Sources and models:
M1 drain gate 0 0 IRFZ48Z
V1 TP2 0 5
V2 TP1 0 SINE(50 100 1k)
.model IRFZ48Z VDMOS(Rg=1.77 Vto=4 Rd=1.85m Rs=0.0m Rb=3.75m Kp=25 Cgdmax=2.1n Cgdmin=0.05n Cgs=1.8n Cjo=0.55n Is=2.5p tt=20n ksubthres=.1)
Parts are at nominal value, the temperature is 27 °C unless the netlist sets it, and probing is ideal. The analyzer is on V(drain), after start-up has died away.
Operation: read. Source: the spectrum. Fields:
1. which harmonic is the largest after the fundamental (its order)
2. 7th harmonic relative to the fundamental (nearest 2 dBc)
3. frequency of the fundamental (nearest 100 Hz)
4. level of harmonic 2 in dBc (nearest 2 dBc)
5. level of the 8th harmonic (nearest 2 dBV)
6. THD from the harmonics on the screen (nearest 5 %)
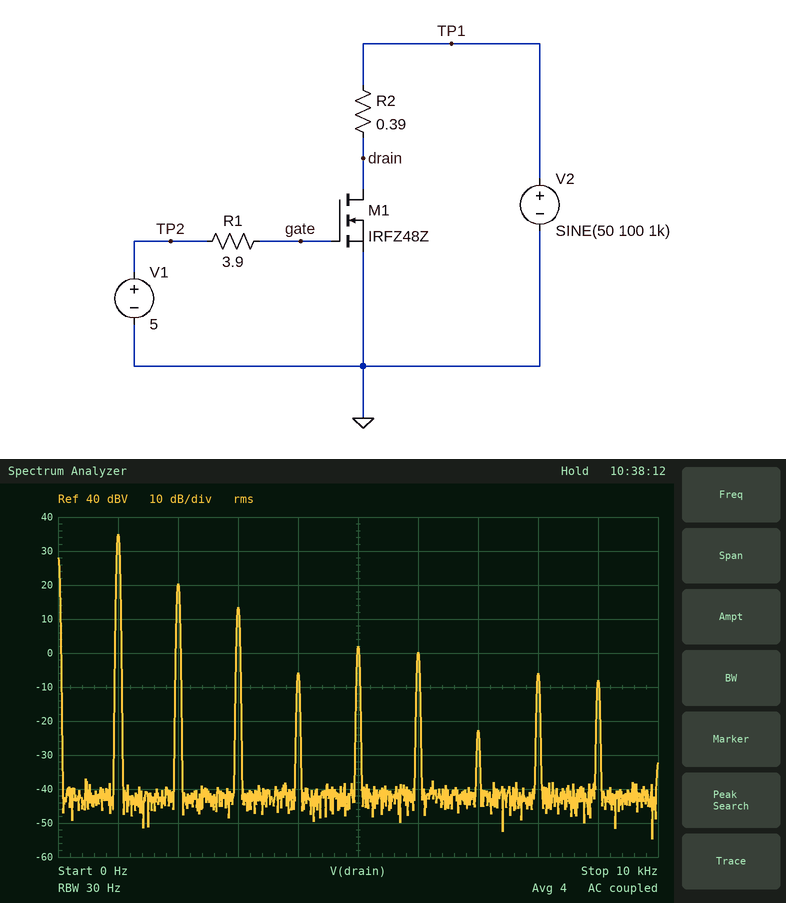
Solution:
2
-58 dBc
1.0 kHz
-14 dBc
-6 dBV
20 %
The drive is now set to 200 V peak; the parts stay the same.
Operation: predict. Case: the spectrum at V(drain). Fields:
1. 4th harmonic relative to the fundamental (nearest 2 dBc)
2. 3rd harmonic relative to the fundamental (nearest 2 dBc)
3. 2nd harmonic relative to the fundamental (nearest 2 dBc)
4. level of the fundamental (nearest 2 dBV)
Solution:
-28 dBc
-24 dBc
-10 dBc
40 dBV
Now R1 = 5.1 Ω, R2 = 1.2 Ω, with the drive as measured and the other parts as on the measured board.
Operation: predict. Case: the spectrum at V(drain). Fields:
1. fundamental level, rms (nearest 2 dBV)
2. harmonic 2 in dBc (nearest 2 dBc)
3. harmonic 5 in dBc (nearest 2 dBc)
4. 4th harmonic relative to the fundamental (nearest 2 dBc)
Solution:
34 dBV
-12 dBc
-30 dBc
-38 dBc
